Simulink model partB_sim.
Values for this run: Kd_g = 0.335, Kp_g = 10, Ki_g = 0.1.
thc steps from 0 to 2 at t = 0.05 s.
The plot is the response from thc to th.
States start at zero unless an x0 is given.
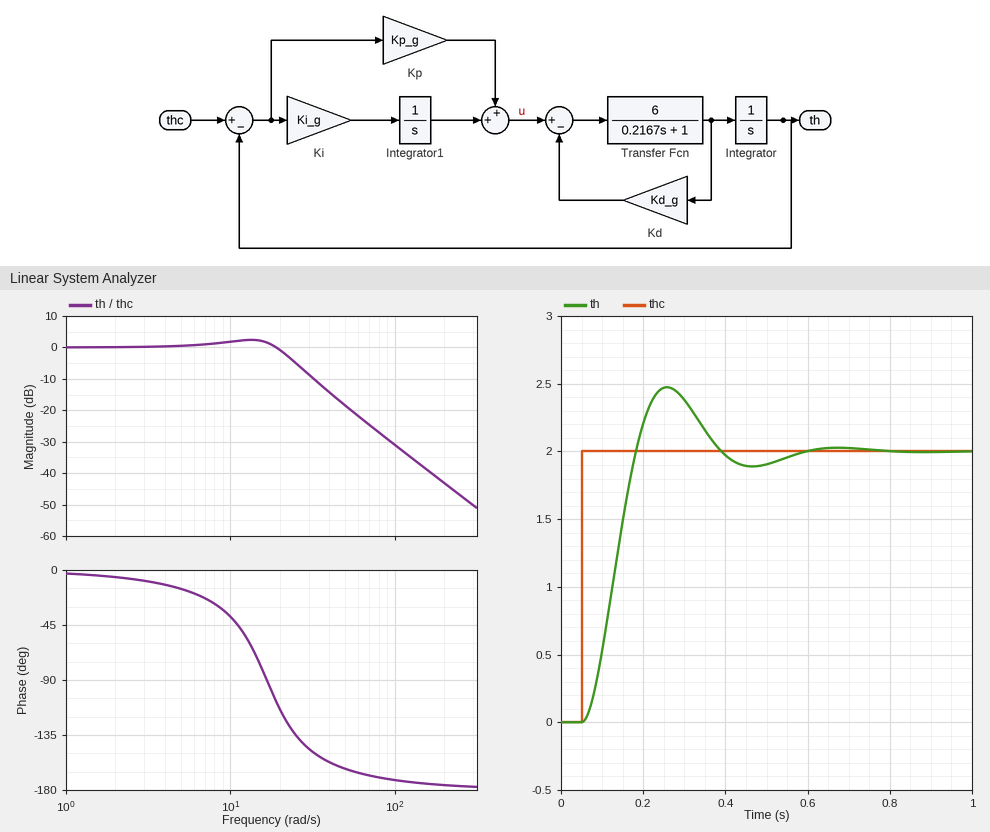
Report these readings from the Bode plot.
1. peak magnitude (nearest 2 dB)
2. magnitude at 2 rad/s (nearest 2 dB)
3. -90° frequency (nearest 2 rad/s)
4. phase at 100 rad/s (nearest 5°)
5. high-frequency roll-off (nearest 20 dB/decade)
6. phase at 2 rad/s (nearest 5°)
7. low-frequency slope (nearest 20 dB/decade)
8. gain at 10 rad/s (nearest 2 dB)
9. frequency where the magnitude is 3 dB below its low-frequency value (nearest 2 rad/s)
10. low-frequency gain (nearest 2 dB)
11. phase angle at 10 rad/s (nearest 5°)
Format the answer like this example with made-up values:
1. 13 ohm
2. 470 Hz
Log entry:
1. 2 dB
2. 0 dB
3. 16 rad/s
4. -170°
5. -40 dB/decade
6. -5°
7. 0 dB/decade
8. 2 dB
9. 22 rad/s
10. 0 dB
11. -40°
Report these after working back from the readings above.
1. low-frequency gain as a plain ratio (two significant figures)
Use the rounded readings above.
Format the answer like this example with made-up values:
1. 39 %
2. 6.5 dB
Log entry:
1. 1.0
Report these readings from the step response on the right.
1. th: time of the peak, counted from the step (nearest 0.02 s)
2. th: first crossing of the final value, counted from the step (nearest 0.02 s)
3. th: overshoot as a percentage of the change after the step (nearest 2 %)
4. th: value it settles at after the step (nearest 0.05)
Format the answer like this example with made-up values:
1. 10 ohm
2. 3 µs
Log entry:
1. 0.20 s
2. 0.14 s
3. 24 %
4. 2.00
